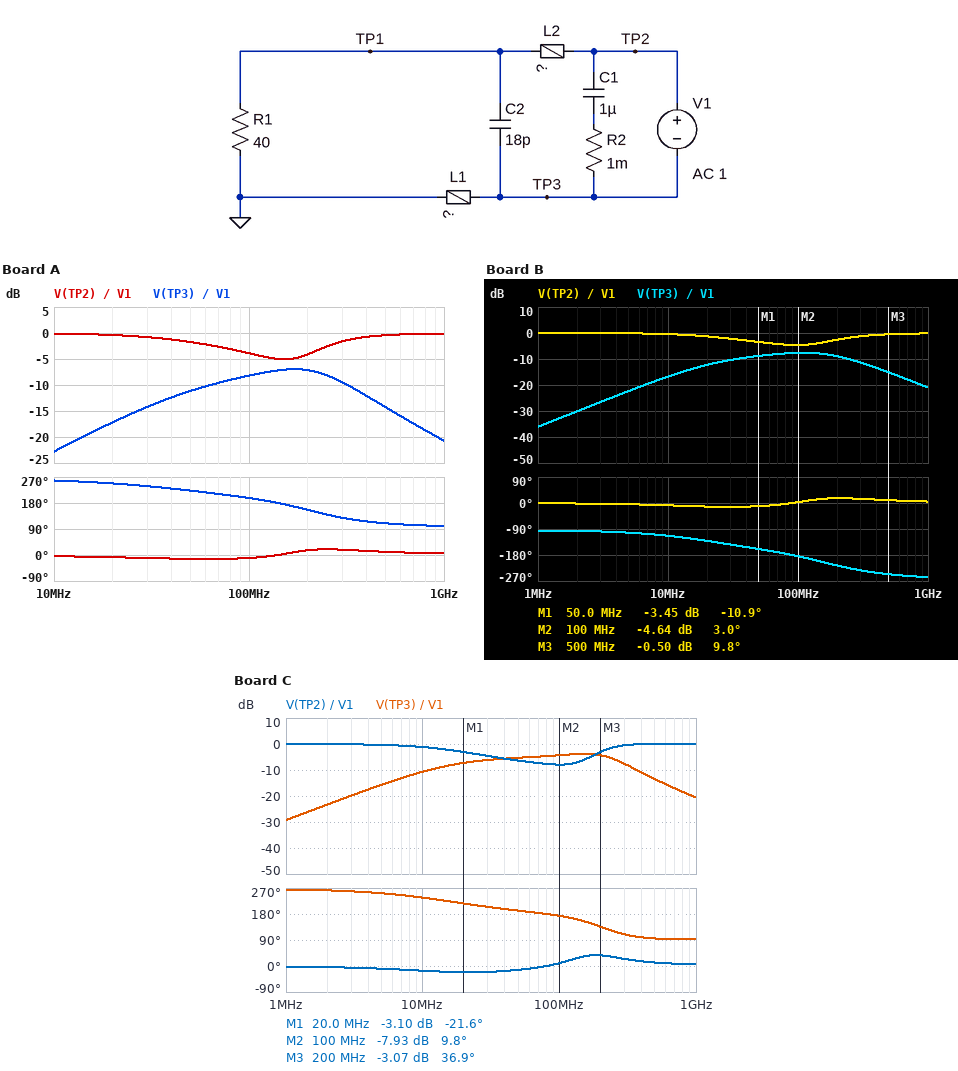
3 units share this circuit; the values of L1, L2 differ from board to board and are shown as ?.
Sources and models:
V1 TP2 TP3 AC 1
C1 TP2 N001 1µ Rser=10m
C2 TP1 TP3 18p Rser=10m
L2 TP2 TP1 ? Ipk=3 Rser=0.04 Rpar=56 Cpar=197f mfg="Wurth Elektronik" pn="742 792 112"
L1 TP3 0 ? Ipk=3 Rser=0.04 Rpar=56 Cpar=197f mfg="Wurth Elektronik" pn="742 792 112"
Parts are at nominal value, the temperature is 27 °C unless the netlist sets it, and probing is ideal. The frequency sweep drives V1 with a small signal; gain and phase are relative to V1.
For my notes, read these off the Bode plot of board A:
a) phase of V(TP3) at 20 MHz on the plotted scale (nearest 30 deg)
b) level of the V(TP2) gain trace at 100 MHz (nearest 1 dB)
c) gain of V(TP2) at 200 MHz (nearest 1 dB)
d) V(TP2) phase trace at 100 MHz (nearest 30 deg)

240 deg
-4 dB
-4 dB
0 deg
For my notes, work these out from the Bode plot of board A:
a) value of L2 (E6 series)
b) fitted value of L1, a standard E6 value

47 nH
47 nH
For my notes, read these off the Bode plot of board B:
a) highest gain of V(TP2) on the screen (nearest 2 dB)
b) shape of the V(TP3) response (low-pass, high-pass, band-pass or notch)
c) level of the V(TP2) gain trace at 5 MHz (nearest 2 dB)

0 dB
band-pass
0 dB
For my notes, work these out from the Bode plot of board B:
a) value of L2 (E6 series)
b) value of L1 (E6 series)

100 nH
100 nH
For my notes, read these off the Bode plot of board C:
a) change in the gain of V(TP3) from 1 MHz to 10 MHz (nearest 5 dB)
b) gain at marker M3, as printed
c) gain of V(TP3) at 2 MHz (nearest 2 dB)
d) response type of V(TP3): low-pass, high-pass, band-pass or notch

20 dB
-3.07 dB
-24 dB
band-pass
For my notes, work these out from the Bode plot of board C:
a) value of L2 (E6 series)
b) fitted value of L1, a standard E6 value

33 nH
220 nH
